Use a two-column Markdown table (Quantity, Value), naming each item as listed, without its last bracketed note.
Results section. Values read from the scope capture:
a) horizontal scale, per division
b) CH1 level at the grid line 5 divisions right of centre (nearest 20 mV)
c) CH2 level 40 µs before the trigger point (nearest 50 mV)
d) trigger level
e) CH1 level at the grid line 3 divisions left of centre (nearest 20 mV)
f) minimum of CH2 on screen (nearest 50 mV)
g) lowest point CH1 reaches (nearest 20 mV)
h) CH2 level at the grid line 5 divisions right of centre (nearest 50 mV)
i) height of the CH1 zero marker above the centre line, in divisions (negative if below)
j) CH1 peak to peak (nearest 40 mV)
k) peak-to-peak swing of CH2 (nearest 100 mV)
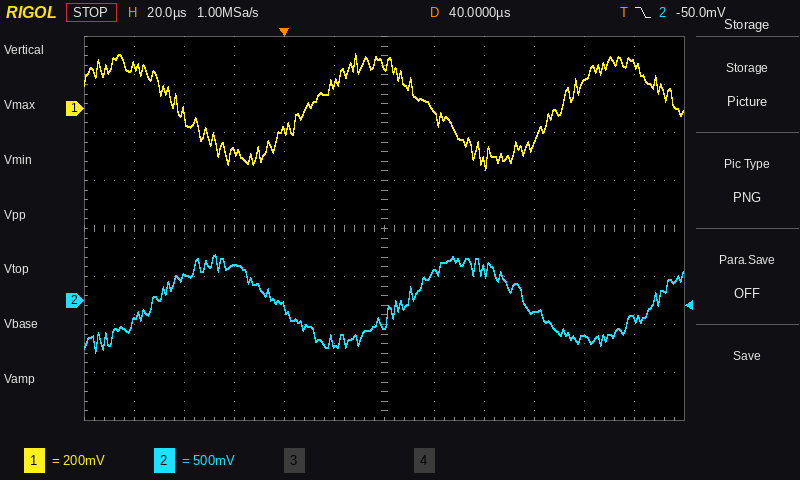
| Quantity | Value |
|---|---|
| horizontal scale, per division | 20 µs |
| CH1 level at the grid line 5 divisions right of centre | 180 mV |
| CH2 level 40 µs before the trigger point | 250 mV |
| trigger level | -50.0 mV |
| CH1 level at the grid line 3 divisions left of centre | -180 mV |
| minimum of CH2 on screen | -550 mV |
| lowest point CH1 reaches | -260 mV |
| CH2 level at the grid line 5 divisions right of centre | -200 mV |
| height of the CH1 zero marker above the centre line, in divisions | +2.5 div |
| CH1 peak to peak | 480 mV |
| peak-to-peak swing of CH2 | 1.00 V |
